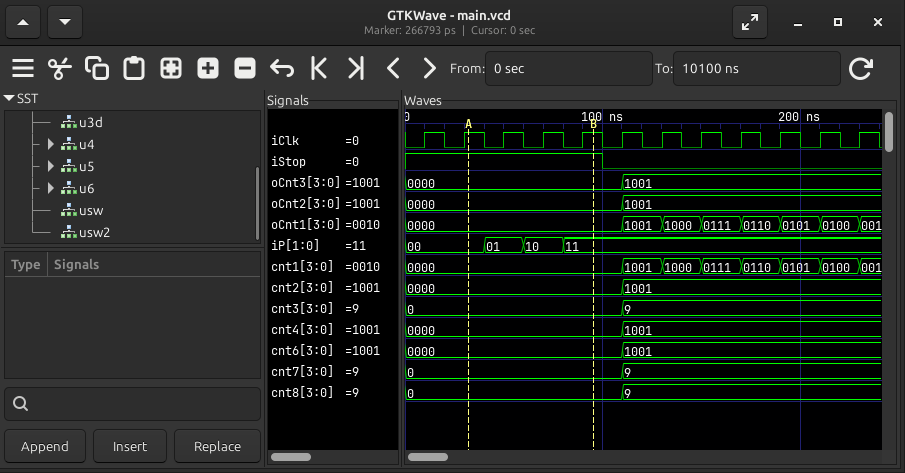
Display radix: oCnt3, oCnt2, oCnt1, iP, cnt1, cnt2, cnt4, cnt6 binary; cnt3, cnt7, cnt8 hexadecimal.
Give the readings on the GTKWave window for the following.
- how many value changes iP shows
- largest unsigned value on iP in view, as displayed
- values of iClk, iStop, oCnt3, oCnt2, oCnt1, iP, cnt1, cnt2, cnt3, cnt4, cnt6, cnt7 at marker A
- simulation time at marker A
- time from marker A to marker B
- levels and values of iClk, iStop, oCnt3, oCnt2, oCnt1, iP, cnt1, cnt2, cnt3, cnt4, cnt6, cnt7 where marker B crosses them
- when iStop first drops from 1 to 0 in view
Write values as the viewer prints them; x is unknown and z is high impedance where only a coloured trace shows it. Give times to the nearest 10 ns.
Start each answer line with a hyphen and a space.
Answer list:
- 3
- 11
- iClk=1, iStop=1, oCnt3=0000, oCnt2=0000, oCnt1=0000, iP=00, cnt1=0000, cnt2=0000, cnt3=0, cnt4=0000, cnt6=0000, cnt7=0
- 30 ns
- 60 ns
- iClk=1, iStop=1, oCnt3=0000, oCnt2=0000, oCnt1=0000, iP=11, cnt1=0000, cnt2=0000, cnt3=0, cnt4=0000, cnt6=0000, cnt7=0
- 100 ns
